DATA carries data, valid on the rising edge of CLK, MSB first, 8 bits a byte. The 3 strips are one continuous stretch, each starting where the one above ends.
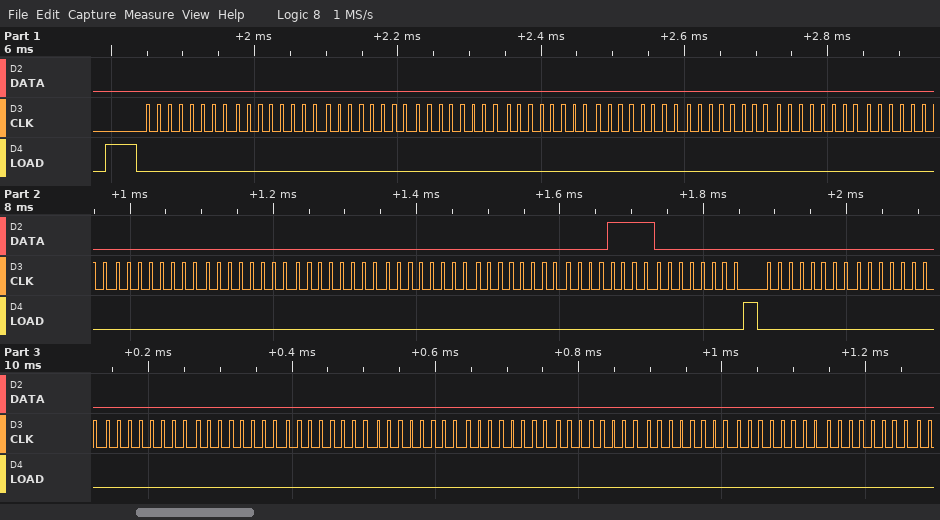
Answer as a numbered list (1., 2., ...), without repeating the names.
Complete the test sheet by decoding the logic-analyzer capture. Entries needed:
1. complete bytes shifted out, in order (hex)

1. 00 00 00 00 00 00 00 00 00 00 00 00 00 00 0F 00 00 00 00 00 00 00 00 00 00 00 00
